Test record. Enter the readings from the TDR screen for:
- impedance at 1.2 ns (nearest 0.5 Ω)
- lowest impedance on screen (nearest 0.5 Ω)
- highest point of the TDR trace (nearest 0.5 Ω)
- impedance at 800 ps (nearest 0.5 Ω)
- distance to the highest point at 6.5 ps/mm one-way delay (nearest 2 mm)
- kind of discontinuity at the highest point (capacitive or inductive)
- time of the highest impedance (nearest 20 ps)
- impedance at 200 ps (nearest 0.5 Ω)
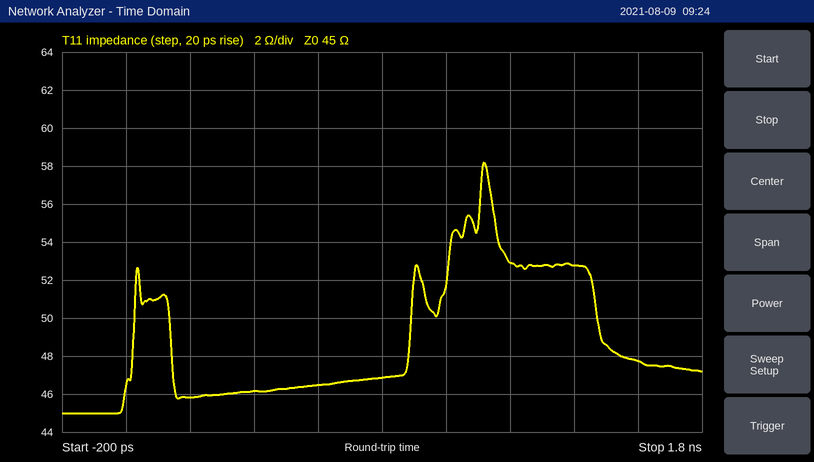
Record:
53.0 Ω
45.0 Ω
58.0 Ω
47.0 Ω
86 mm
inductive
1.12 ns
46.0 Ω
